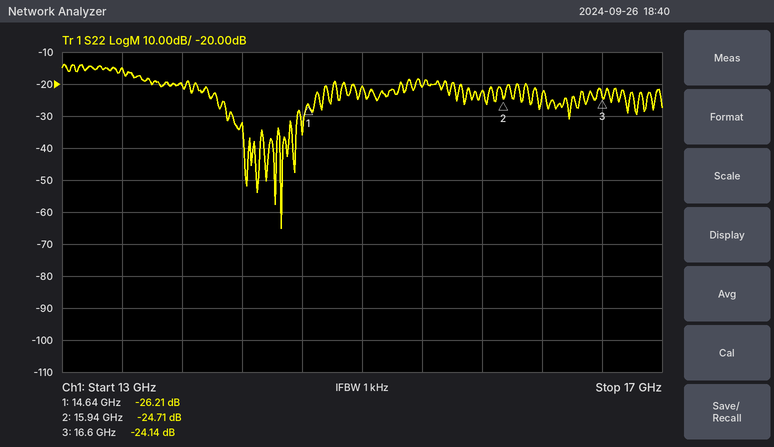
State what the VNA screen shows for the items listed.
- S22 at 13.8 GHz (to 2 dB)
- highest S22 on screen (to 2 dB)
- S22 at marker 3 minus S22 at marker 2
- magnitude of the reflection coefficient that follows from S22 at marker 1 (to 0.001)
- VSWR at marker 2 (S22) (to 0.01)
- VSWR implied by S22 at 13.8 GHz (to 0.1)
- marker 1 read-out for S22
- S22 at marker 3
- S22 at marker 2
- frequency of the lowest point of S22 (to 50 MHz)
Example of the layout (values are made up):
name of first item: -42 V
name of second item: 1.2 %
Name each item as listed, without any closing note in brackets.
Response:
S22 at 13.8 GHz: -20 dB
highest S22 on screen: -14 dB
S22 at marker 3 minus S22 at marker 2: 0.57 dB
magnitude of the reflection coefficient that follows from S22 at marker 1: 0.049
VSWR at marker 2 (S22): 1.12
VSWR implied by S22 at 13.8 GHz: 1.2
marker 1 read-out for S22: -26.21 dB
S22 at marker 3: -24.14 dB
S22 at marker 2: -24.71 dB
frequency of the lowest point of S22: 14.45 GHz
